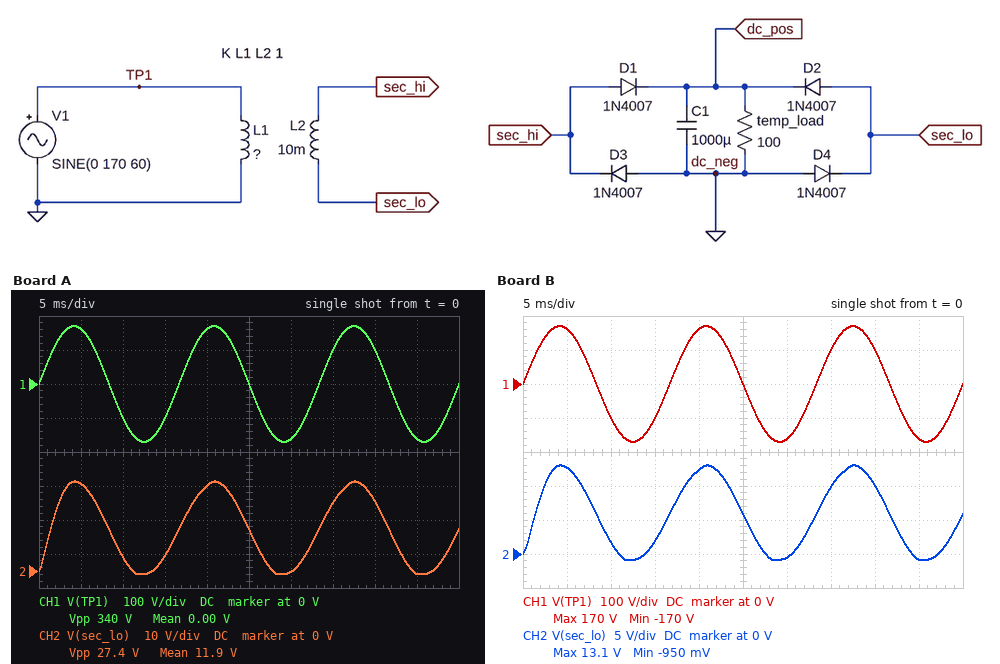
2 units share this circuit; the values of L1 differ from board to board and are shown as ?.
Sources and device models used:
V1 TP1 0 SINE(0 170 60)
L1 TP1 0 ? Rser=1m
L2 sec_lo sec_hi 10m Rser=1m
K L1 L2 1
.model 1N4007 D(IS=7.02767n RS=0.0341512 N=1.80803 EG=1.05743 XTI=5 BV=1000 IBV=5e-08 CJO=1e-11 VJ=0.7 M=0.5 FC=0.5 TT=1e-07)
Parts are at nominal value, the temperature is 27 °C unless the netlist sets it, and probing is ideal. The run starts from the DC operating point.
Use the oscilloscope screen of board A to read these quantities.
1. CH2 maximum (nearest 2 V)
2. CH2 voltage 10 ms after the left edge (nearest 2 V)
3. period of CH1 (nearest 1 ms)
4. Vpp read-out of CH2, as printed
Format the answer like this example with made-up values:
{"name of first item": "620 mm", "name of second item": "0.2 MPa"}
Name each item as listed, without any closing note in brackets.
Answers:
{"CH2 maximum": "26 V", "CH2 voltage 10 ms after the left edge": "4 V", "period of CH1": "17 ms", "Vpp read-out of CH2, as printed": "27.4 V"}
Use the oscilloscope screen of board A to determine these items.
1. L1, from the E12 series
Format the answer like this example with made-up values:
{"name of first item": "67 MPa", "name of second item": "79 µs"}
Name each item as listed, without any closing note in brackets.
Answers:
{"L1, from the E12 series": "390 mH"}
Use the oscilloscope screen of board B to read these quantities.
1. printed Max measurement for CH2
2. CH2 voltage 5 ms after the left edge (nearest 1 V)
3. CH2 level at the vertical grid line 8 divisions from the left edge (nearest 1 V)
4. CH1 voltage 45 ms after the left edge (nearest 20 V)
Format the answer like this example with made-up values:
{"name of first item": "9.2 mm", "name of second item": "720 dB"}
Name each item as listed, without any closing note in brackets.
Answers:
{"printed Max measurement for CH2": "13.1 V", "CH2 voltage 5 ms after the left edge": "13 V", "CH2 level at the vertical grid line 8 divisions from the left edge": "10 V", "CH1 voltage 45 ms after the left edge": "-160 V"}
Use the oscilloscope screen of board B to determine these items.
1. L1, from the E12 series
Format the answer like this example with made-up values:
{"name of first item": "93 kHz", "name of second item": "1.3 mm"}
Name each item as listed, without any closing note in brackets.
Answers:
{"L1, from the E12 series": "1.5 H"}
